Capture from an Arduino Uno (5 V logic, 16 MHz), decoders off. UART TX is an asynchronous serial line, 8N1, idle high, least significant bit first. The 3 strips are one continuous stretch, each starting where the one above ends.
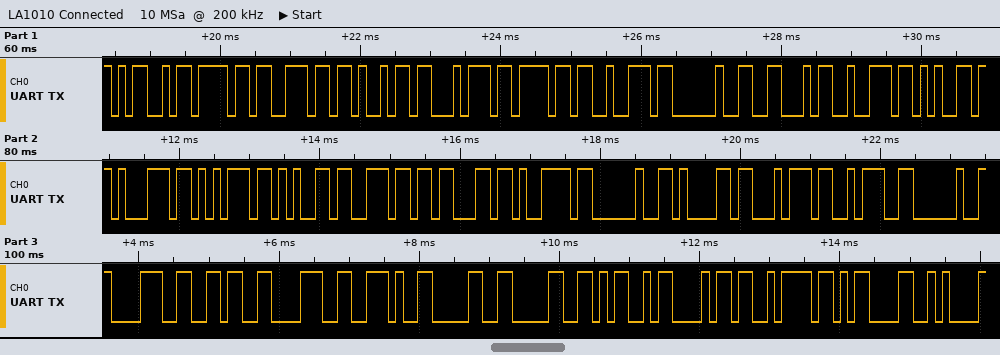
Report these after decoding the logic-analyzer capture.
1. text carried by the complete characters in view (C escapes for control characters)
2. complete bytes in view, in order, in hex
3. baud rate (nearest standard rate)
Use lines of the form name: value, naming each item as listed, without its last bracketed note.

text carried by the complete characters in view: "Monitor Frequency at: 868.00Mhz\r\n"
complete bytes in view, in order, in hex: 0x4D 0x6F 0x6E 0x69 0x74 0x6F 0x72 0x20 0x46 0x72 0x65 0x71 0x75 0x65 0x6E 0x63 0x79 0x20 0x61 0x74 0x3A 0x20 0x38 0x36 0x38 0x2E 0x30 0x30 0x4D 0x68 0x7A 0x0D 0x0A
baud rate: 9600 baud
